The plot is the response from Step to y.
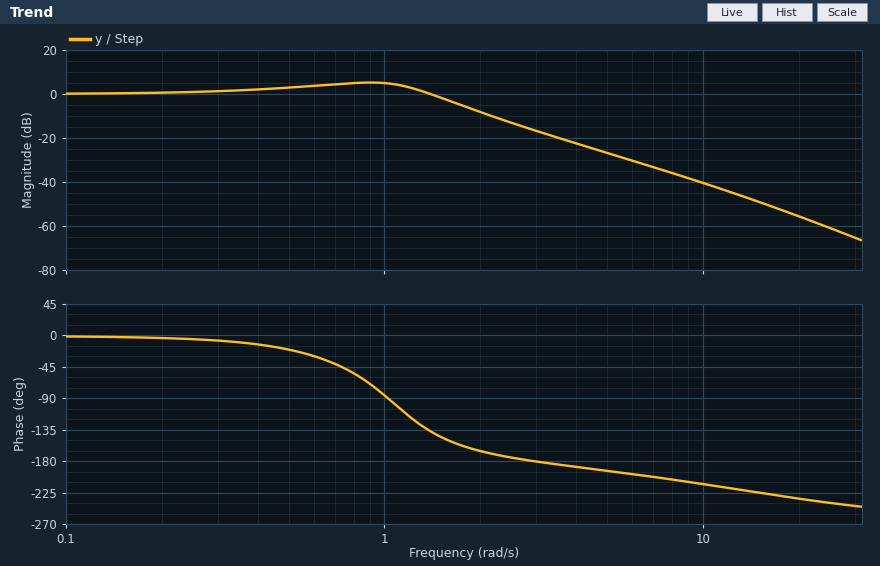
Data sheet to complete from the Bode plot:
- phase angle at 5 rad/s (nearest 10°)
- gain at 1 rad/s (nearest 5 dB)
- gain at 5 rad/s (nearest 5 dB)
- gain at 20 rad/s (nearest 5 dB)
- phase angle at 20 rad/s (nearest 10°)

-190°
5 dB
-25 dB
-55 dB
-230°
